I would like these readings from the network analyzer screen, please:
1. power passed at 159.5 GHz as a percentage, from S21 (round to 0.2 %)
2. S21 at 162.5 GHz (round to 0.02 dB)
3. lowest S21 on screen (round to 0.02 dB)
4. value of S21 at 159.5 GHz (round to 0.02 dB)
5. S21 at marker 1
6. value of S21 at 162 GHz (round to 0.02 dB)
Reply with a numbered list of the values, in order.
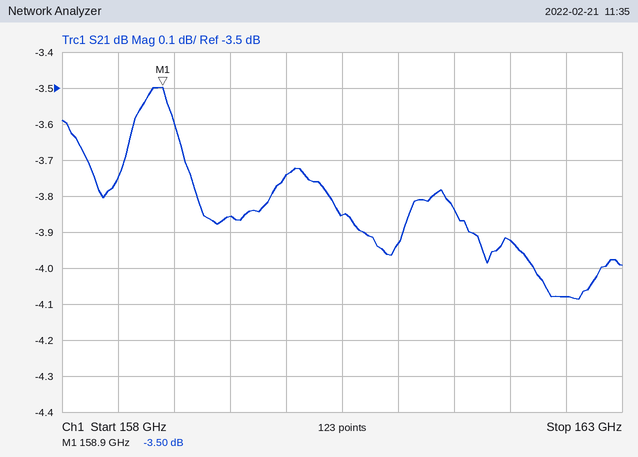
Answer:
1. 41.2 %
2. -4.08 dB
3. -4.08 dB
4. -3.86 dB
5. -3.50 dB
6. -3.92 dB
